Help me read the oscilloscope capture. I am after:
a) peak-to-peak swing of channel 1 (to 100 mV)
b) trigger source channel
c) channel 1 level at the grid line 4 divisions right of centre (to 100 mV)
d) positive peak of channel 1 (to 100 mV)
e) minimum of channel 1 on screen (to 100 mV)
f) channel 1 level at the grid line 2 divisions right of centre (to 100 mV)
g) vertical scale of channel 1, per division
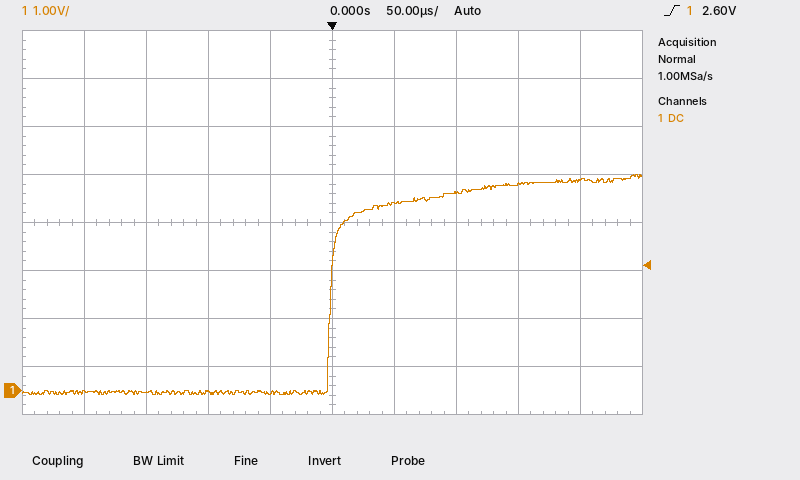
4.6 V
channel 1
4.4 V
4.5 V
-100 mV
4.1 V
1 V
